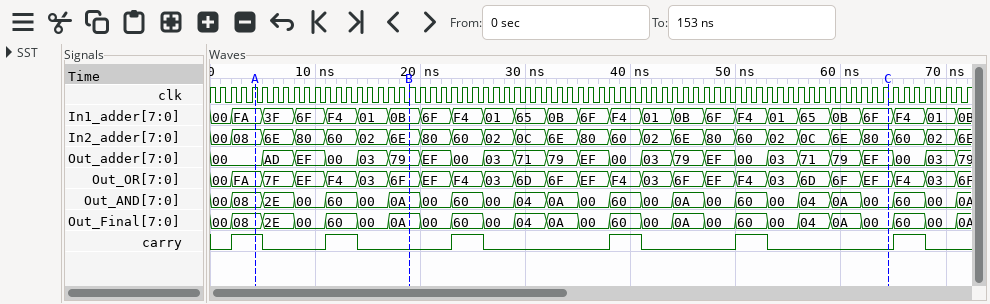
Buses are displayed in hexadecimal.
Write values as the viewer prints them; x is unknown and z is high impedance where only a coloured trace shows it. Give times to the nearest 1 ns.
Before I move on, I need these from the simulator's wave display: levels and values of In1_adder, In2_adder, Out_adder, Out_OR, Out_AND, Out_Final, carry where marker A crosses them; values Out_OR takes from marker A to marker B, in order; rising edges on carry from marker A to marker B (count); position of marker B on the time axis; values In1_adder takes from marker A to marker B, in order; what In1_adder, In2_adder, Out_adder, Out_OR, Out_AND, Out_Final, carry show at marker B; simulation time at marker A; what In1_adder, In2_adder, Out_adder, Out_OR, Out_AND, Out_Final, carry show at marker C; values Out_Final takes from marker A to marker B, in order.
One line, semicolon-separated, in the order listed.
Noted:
In1_adder=FA, In2_adder=08, Out_adder=00, Out_OR=FA, Out_AND=08, Out_Final=08, carry=1; FA, 7F, EF, F4, 03, 6F; 1; 19 ns; FA, 3F, 6F, F4, 01, 0B; In1_adder=0B, In2_adder=6E, Out_adder=79, Out_OR=6F, Out_AND=0A, Out_Final=0A, carry=0; 4 ns; In1_adder=6F, In2_adder=80, Out_adder=EF, Out_OR=EF, Out_AND=00, Out_Final=00, carry=0; 08, 2E, 00, 60, 00, 0A
